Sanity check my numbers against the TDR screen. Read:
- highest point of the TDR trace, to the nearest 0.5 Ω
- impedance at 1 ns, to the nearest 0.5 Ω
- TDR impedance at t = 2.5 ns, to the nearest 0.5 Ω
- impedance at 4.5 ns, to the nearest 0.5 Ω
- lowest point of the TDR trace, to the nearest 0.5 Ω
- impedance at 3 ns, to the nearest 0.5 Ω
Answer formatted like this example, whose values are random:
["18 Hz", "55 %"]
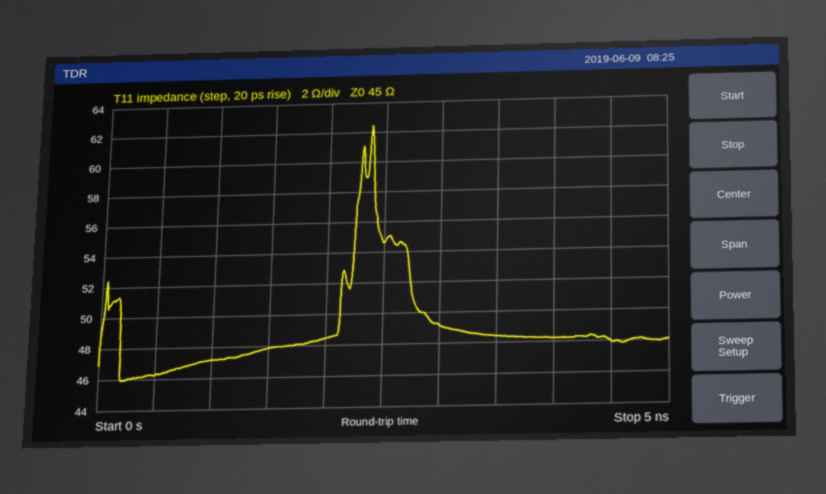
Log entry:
["62.5 Ω", "47.0 Ω", "54.5 Ω", "48.0 Ω", "46.0 Ω", "49.0 Ω"]
